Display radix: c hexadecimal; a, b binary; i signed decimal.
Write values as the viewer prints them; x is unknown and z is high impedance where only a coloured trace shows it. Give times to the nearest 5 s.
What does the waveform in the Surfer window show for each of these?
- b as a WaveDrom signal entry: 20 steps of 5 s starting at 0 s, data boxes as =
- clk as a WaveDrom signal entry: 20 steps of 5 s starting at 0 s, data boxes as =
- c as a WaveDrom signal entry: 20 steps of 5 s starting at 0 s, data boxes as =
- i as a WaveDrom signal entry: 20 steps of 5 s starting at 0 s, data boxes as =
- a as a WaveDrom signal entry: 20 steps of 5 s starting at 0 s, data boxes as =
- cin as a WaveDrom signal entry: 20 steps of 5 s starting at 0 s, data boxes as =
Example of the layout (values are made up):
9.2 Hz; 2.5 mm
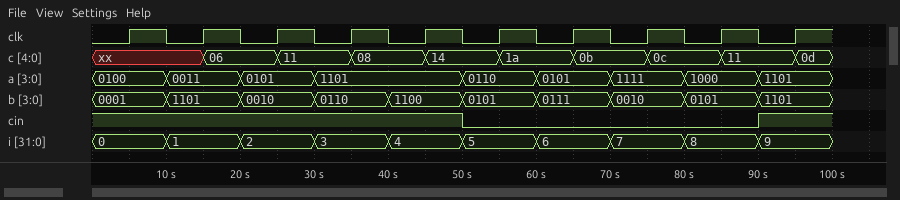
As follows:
{name: 'b', wave: '=.=.=.=.=.=.=.=.=.=.', data: '0001 1101 0010 0110 1100 0101 0111 0010 0101 1101'}; {name: 'clk', wave: '01010101010101010101'}; {name: 'c', wave: 'x..=.=.=.=.=.=.=.=.=', data: '06 11 08 14 1a 0b 0c 11 0d'}; {name: 'i', wave: '=.=.=.=.=.=.=.=.=.=.', data: '0 1 2 3 4 5 6 7 8 9'}; {name: 'a', wave: '=.=.=.=...=.=.=.=.=.', data: '0100 0011 0101 1101 0110 0101 1111 1000 1101'}; {name: 'cin', wave: '1.........0.......1.'}
